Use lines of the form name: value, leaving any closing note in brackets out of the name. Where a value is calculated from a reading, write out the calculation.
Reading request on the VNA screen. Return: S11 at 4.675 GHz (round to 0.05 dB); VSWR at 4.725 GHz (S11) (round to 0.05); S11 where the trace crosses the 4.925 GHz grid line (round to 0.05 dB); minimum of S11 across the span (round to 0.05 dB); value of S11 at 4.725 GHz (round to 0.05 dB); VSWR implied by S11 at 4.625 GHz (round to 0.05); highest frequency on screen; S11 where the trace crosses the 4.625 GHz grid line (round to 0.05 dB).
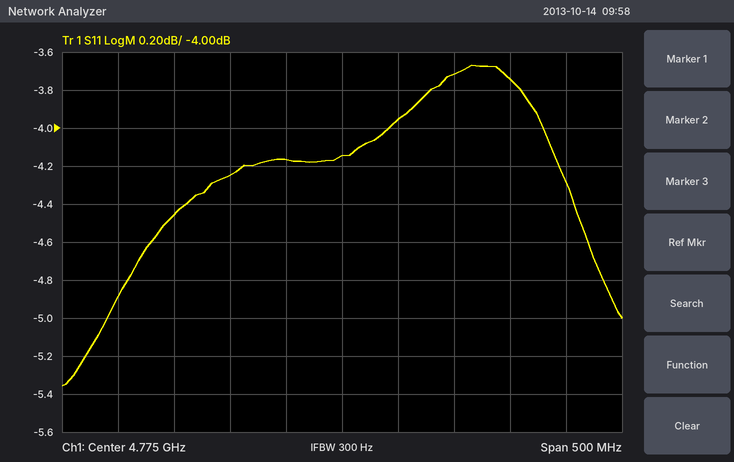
S11 at 4.675 GHz: -4.25 dB
VSWR at 4.725 GHz (S11): |Γ| = 10^(-4.15/20) = 0.6202; VSWR = (1 + 0.6202)/(1 − 0.6202) ≈ 4.27, so 4.25 to the nearest 0.05
S11 where the trace crosses the 4.925 GHz grid line: -3.75 dB
minimum of S11 across the span: -5.35 dB
value of S11 at 4.725 GHz: -4.15 dB
VSWR implied by S11 at 4.625 GHz: |Γ| = 10^(-4.45/20) = 0.5991; VSWR = (1 + 0.5991)/(1 − 0.5991) ≈ 3.99, so 4.00 to the nearest 0.05
highest frequency on screen: 5.025 GHz
S11 where the trace crosses the 4.625 GHz grid line: -4.45 dB
